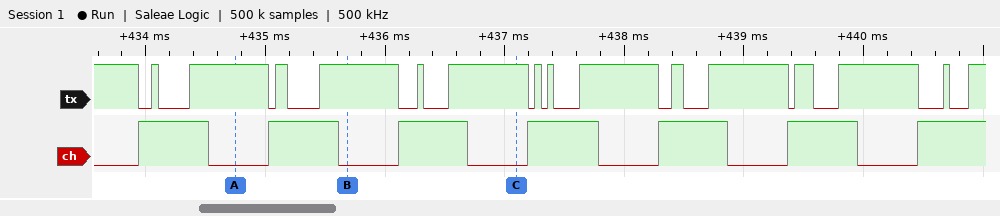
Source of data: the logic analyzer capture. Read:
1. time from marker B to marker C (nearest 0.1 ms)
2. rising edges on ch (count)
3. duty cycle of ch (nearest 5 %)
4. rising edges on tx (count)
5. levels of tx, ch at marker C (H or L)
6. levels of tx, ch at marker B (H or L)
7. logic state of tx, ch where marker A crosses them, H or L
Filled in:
1.4 ms
7
55 %
15
tx=H, ch=L
tx=H, ch=L
tx=H, ch=L
